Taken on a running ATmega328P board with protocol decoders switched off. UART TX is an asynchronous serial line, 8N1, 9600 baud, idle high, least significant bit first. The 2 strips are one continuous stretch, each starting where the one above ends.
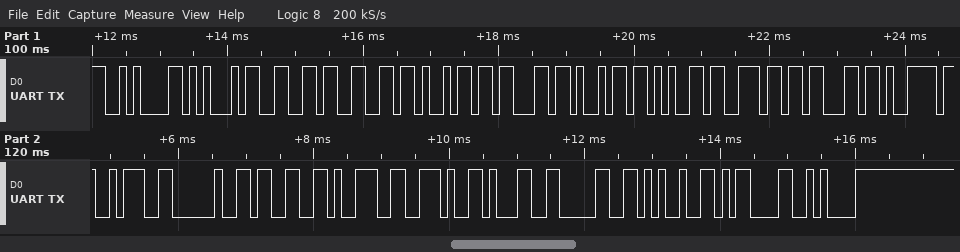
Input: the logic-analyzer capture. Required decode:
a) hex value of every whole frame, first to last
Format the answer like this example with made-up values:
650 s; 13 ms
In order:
0A 45 66 66 69 63 69 65 6E 63 79 3A 20 33 39 2E 31 30 25 0D 0A
